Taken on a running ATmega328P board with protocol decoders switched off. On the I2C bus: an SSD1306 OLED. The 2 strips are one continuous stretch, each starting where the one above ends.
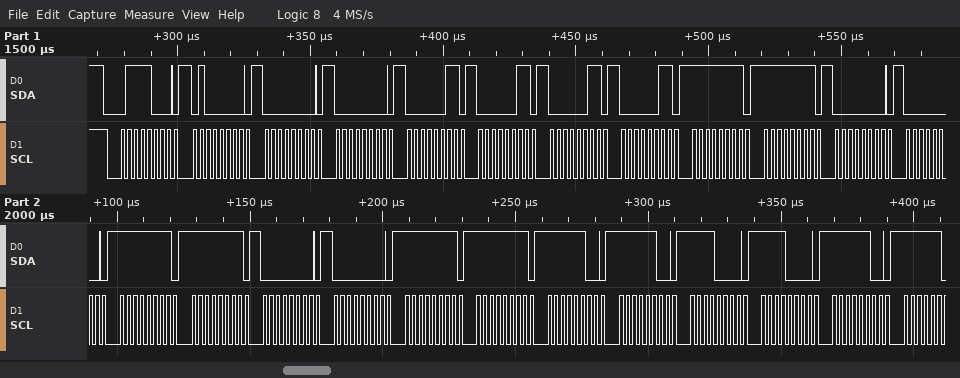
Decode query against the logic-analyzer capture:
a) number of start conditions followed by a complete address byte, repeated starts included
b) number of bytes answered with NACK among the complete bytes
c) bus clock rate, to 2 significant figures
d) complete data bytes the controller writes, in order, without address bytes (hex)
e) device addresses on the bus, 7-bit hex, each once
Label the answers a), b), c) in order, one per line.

a) 1
b) 0
c) 400 kHz
d) 40 00 00 03 03 03 03 FF FF 00 00 FF FF 00 00 FF FF FC FC F0 F0 FC
e) 0x3C
